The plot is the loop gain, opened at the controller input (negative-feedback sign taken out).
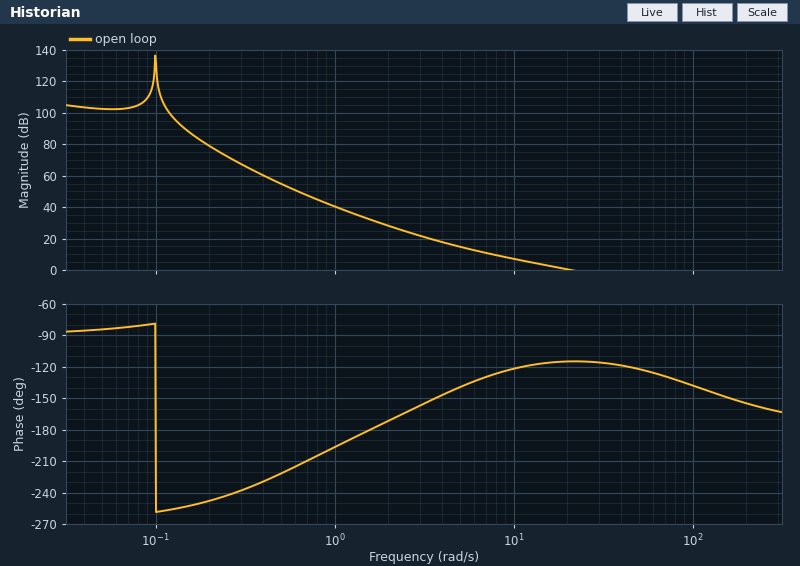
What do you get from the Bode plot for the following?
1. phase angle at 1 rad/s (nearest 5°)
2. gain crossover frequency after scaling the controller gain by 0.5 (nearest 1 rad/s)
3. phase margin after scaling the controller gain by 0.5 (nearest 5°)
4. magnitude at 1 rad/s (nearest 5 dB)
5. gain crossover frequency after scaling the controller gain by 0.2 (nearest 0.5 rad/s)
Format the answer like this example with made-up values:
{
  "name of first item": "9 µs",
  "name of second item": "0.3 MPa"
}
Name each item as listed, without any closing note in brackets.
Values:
{
  "phase angle at 1 rad/s": "-195°",
  "gain crossover frequency after scaling the controller gain by 0.5": "11 rad/s",
  "phase margin after scaling the controller gain by 0.5": "60°",
  "magnitude at 1 rad/s": "40 dB",
  "gain crossover frequency after scaling the controller gain by 0.2": "5.5 rad/s"
}
